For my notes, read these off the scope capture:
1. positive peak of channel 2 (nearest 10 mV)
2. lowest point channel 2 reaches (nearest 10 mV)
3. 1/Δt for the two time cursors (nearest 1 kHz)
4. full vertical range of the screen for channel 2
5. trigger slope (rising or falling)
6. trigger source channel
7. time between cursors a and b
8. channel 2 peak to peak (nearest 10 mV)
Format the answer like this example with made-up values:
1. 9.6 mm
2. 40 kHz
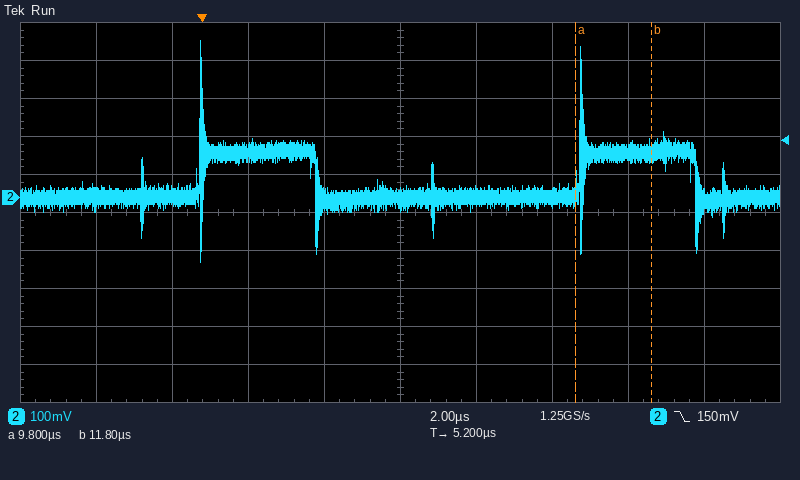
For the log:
1. 410 mV
2. -170 mV
3. 500 kHz
4. 1 V
5. falling
6. channel 2
7. 2.0 µs
8. 580 mV
